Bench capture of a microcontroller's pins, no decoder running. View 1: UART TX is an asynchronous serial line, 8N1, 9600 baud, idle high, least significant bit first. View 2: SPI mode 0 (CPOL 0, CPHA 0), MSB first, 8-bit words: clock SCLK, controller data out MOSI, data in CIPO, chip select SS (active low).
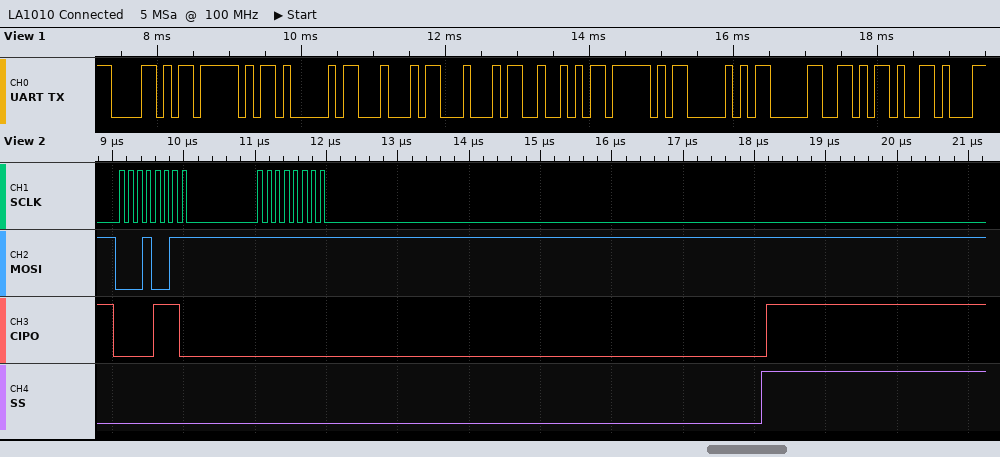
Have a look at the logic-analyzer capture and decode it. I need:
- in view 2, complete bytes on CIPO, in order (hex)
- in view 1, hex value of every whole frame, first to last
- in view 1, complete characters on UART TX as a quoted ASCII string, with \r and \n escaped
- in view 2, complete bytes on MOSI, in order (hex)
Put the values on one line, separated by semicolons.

0E 00; 58 5F 41 44 44 52 5F 50 30 2D; "X_ADDR_P0-"; 13 FF
